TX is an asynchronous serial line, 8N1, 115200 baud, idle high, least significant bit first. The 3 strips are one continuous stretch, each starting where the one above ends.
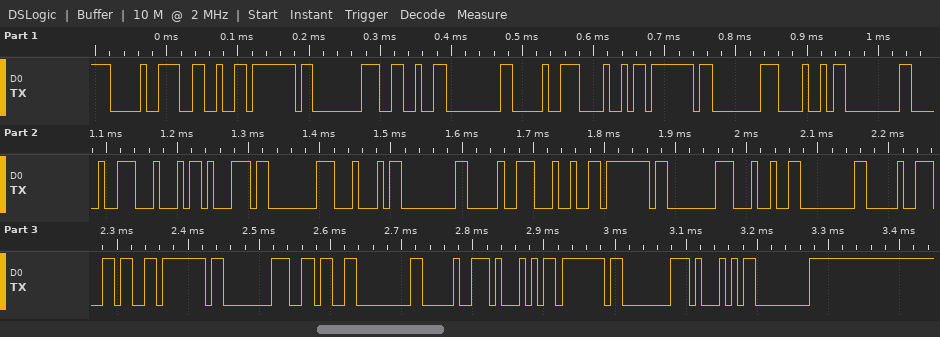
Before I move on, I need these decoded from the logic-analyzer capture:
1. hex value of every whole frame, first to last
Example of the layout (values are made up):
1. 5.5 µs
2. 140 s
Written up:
1. 90 26 7F 80 26 00 90 48 7F 80 48 00 90 44 71 80 44 00 90 24 7F 80 24 00 90 36 7F 80 36 00 90 51 7F 80 51 00
